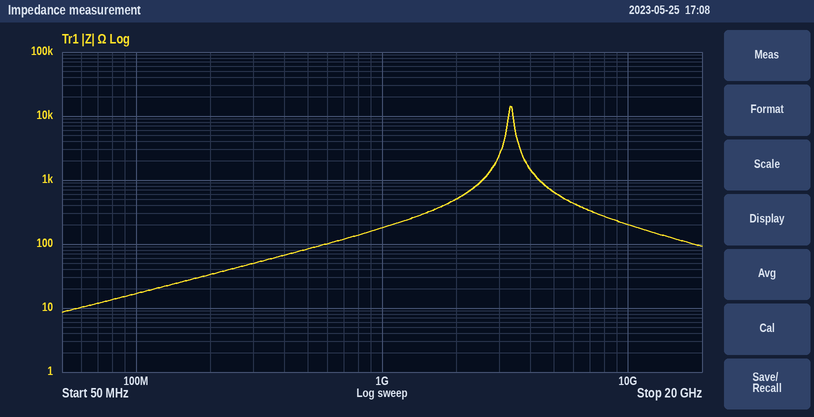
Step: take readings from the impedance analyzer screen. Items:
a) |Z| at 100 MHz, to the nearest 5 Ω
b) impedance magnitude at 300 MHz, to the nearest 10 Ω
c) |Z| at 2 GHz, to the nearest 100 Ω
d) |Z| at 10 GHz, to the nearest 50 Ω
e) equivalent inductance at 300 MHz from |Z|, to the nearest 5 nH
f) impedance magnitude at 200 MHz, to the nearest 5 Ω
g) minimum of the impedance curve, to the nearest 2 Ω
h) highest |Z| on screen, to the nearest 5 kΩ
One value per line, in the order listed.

15 Ω
50 Ω
500 Ω
200 Ω
25 nH
35 Ω
8 Ω
15 kΩ
